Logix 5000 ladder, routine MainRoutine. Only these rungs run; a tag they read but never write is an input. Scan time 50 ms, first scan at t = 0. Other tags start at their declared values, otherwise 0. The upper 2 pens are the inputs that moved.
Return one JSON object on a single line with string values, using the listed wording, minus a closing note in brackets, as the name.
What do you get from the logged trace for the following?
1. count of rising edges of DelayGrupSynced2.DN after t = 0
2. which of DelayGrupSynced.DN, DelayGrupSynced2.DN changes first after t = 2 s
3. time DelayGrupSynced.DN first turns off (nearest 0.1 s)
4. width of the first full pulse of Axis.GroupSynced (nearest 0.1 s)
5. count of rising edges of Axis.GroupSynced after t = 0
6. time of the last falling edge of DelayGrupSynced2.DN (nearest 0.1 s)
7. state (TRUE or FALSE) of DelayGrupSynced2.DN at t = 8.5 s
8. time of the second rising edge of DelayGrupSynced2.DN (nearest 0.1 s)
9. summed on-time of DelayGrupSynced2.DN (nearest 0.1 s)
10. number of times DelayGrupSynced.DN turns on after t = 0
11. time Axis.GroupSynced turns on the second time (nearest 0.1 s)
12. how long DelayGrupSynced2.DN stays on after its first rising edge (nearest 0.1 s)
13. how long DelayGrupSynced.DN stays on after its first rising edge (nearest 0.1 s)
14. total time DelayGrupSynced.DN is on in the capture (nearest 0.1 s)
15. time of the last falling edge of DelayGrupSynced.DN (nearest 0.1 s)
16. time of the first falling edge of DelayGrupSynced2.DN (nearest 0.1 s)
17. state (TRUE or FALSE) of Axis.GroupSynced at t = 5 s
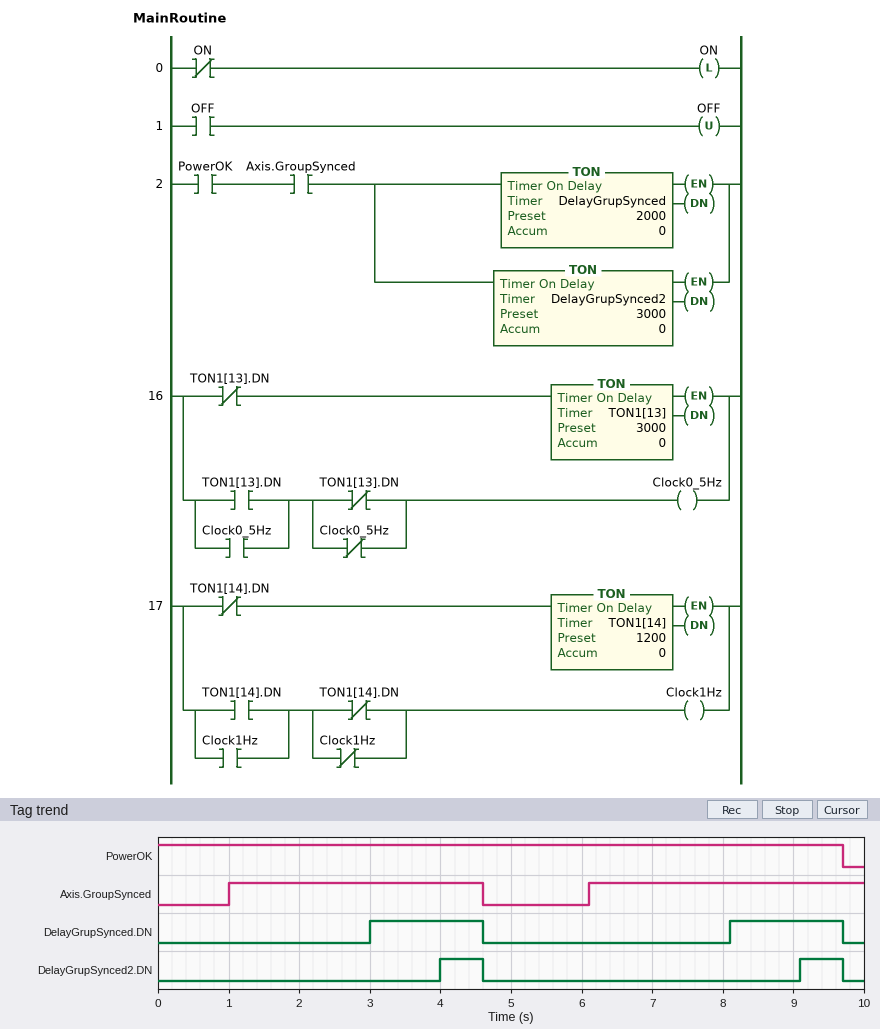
{"count of rising edges of DelayGrupSynced2.DN after t = 0": "2", "which of DelayGrupSynced.DN, DelayGrupSynced2.DN changes first after t = 2 s": "DelayGrupSynced.DN", "time DelayGrupSynced.DN first turns off": "4.6 s", "width of the first full pulse of Axis.GroupSynced": "3.6 s", "count of rising edges of Axis.GroupSynced after t = 0": "2", "time of the last falling edge of DelayGrupSynced2.DN": "9.7 s", "state (TRUE or FALSE) of DelayGrupSynced2.DN at t = 8.5 s": "FALSE", "time of the second rising edge of DelayGrupSynced2.DN": "9.1 s", "summed on-time of DelayGrupSynced2.DN": "1.2 s", "number of times DelayGrupSynced.DN turns on after t = 0": "2", "time Axis.GroupSynced turns on the second time": "6.1 s", "how long DelayGrupSynced2.DN stays on after its first rising edge": "0.6 s", "how long DelayGrupSynced.DN stays on after its first rising edge": "1.6 s", "total time DelayGrupSynced.DN is on in the capture": "3.2 s", "time of the last falling edge of DelayGrupSynced.DN": "9.7 s", "time of the first falling edge of DelayGrupSynced2.DN": "4.6 s", "state (TRUE or FALSE) of Axis.GroupSynced at t = 5 s": "FALSE"}
